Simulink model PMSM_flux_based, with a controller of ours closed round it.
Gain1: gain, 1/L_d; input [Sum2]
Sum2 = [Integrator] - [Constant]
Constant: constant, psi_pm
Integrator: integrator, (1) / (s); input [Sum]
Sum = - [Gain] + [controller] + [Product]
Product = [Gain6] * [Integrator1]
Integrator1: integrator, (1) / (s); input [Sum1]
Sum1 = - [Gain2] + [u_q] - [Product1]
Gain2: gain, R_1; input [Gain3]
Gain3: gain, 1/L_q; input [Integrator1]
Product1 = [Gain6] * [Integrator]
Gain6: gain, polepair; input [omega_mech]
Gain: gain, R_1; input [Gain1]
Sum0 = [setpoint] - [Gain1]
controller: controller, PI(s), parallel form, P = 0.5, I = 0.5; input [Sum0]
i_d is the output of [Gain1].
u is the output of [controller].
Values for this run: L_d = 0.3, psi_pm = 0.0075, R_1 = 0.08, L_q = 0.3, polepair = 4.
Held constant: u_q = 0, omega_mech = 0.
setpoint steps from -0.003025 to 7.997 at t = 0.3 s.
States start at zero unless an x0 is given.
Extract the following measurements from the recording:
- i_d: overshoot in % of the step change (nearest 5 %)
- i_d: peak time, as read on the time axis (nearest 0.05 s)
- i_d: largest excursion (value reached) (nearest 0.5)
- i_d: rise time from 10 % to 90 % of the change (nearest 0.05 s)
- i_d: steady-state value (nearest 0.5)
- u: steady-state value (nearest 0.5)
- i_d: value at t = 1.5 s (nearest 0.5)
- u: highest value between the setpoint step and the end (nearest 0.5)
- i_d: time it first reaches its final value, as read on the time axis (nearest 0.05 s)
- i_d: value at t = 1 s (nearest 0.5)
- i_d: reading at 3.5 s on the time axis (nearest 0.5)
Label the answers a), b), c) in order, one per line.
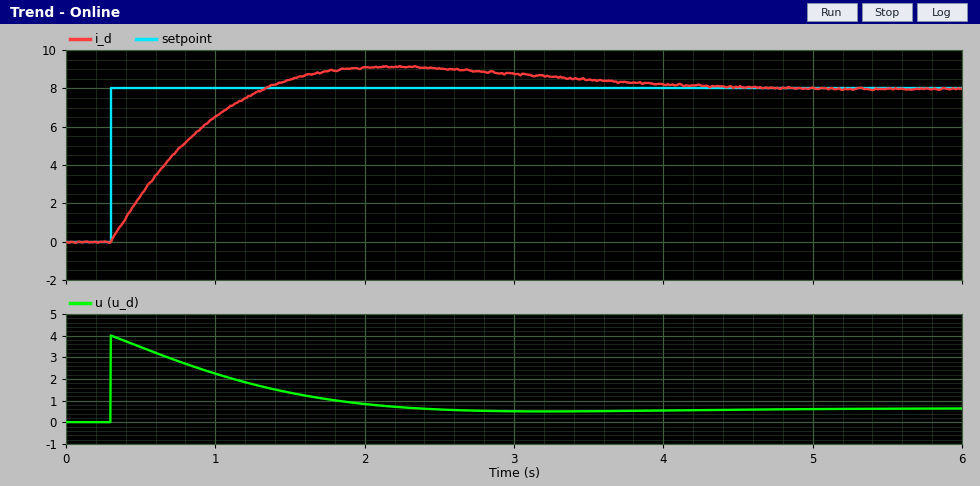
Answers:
a) 15 %
b) 2.20 s
c) 9.0
d) 0.75 s
e) 8.0
f) 0.5
g) 8.5
h) 4.0
i) 1.35 s
j) 6.5
k) 8.5
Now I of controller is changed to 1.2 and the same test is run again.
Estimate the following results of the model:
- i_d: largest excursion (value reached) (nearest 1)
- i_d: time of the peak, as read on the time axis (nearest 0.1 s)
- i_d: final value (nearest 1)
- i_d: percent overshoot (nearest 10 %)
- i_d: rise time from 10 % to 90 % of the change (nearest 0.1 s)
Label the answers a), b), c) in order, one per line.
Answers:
a) 10
b) 1.6 s
c) 8
d) 30 %
e) 0.5 s
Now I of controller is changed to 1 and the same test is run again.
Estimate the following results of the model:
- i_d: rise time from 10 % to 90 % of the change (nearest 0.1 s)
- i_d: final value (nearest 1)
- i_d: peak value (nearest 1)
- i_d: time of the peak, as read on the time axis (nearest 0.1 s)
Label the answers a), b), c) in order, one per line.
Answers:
a) 0.6 s
b) 8
c) 10
d) 1.7 s
